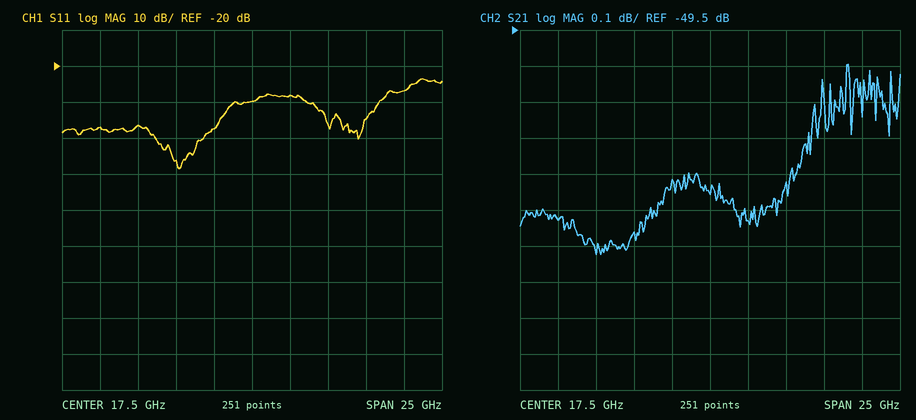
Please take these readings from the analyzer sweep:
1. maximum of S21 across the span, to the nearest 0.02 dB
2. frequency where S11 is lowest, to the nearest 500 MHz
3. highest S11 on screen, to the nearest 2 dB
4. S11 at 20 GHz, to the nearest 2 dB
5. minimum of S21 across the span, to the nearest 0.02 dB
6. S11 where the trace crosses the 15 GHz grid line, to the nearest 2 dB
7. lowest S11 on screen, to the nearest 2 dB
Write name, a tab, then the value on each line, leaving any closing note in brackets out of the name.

maximum of S21 across the span, to the nearest 0.02 dB	-49.60 dB
frequency where S11 is lowest, to the nearest 500 MHz	12.5 GHz
highest S11 on screen, to the nearest 2 dB	-24 dB
S11 at 20 GHz, to the nearest 2 dB	-28 dB
minimum of S21 across the span, to the nearest 0.02 dB	-50.12 dB
S11 where the trace crosses the 15 GHz grid line, to the nearest 2 dB	-38 dB
lowest S11 on screen, to the nearest 2 dB	-48 dB
